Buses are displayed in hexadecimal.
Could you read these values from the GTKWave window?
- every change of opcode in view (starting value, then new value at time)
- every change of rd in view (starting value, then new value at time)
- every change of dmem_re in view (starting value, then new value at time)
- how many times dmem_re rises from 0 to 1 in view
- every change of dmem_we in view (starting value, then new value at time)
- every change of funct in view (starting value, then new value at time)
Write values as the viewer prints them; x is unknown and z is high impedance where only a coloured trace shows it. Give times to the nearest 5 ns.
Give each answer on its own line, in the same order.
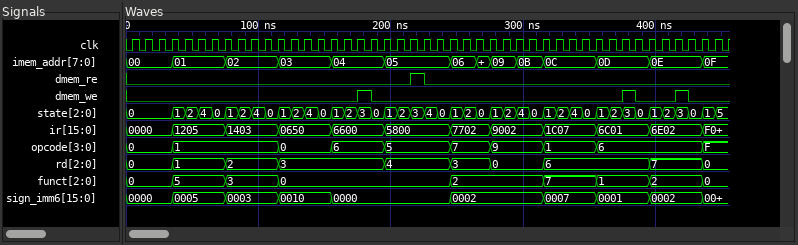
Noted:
0, 1 at 35 ns, 0 at 115 ns, 6 at 155 ns, 5 at 195 ns, 7 at 245 ns, 9 at 275 ns, 1 at 315 ns, 6 at 355 ns, F at 435 ns
0, 1 at 35 ns, 2 at 75 ns, 3 at 115 ns, 4 at 195 ns, 3 at 245 ns, 0 at 275 ns, 6 at 315 ns, 7 at 395 ns, 0 at 435 ns
0, 1 at 215 ns, 0 at 225 ns
1
0, 1 at 175 ns, 0 at 185 ns, 1 at 375 ns, 0 at 385 ns, 1 at 415 ns, 0 at 425 ns
0, 5 at 35 ns, 3 at 75 ns, 0 at 115 ns, 2 at 245 ns, 7 at 315 ns, 1 at 355 ns, 2 at 395 ns, 0 at 435 ns
